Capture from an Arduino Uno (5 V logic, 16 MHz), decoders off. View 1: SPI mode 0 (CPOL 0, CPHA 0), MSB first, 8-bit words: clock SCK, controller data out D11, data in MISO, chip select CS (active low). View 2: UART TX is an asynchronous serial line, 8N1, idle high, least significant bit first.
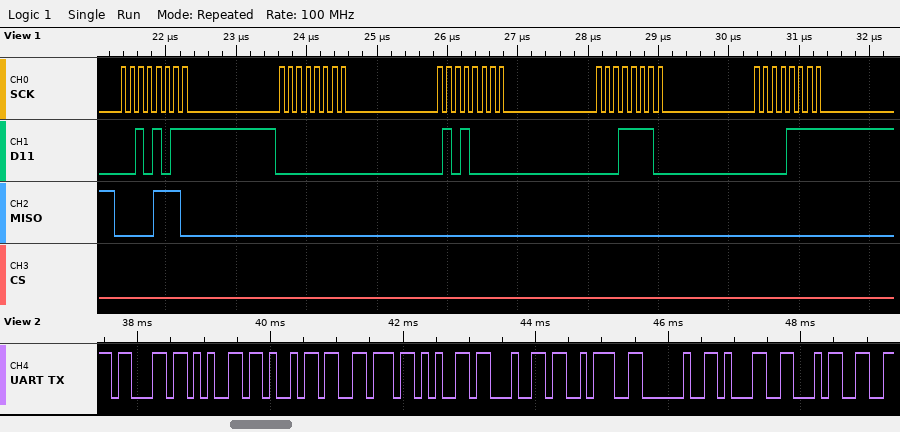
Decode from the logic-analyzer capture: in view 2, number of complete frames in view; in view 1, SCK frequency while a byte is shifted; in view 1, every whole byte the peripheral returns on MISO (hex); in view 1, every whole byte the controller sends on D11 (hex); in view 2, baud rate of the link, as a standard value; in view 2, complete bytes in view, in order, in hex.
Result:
10
8 MHz
0x0E 0x00 0x00 0x00 0x00
0x2B 0x00 0x50 0x1E 0x0F
9600 baud
63 65 69 76 65 64 3A 20 31 34
